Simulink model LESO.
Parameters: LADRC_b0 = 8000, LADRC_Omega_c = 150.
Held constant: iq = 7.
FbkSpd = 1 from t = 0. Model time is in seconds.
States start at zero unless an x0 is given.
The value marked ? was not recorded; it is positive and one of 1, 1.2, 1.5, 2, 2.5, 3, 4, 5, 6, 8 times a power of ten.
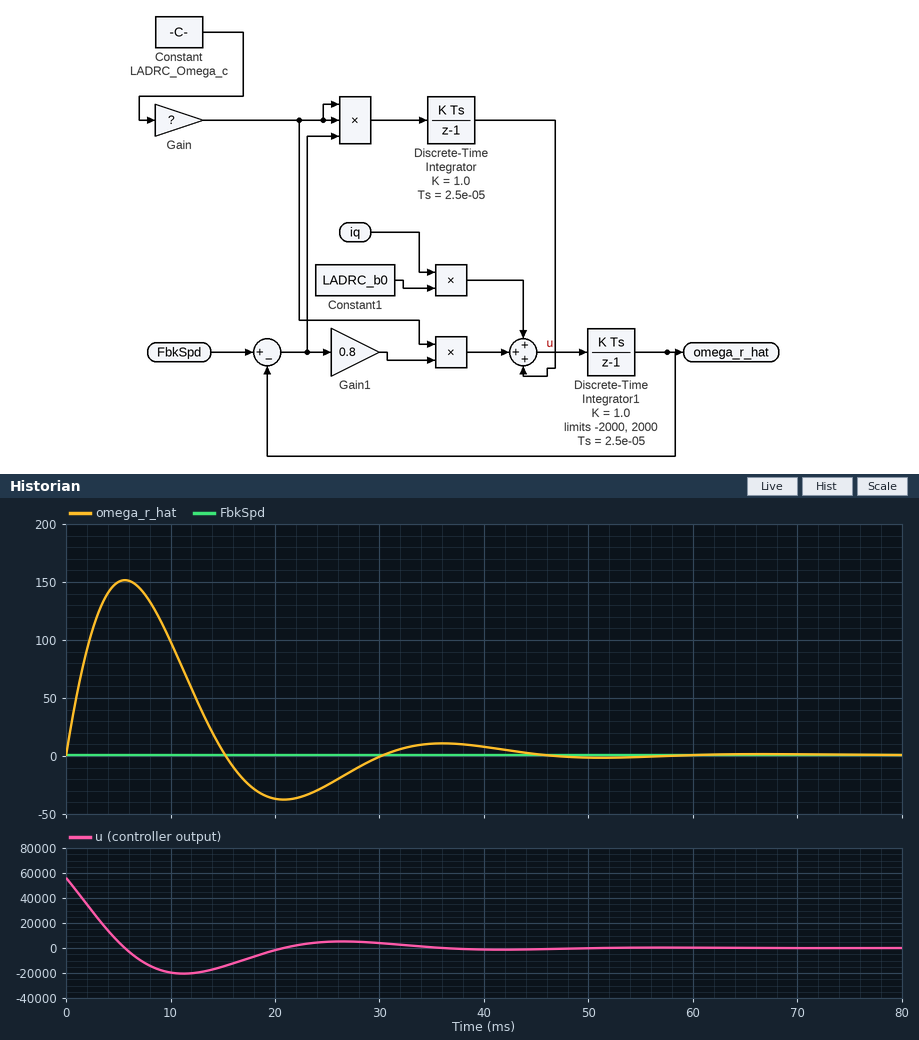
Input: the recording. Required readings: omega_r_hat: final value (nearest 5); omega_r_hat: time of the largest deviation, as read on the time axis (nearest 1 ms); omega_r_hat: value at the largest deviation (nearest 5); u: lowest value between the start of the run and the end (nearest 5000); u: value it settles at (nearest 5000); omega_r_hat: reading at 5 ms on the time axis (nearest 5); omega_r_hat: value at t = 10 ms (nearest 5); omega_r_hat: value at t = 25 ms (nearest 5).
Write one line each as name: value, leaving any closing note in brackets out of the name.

omega_r_hat: final value: 0
omega_r_hat: time of the largest deviation, as read on the time axis: 6 ms
omega_r_hat: value at the largest deviation: 150
u: lowest value between the start of the run and the end: -20000
u: value it settles at: 0
omega_r_hat: reading at 5 ms on the time axis: 150
omega_r_hat: value at t = 10 ms: 100
omega_r_hat: value at t = 25 ms: -25
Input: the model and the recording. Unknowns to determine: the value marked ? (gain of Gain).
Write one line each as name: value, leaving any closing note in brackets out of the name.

the value marked ?: 1.5
